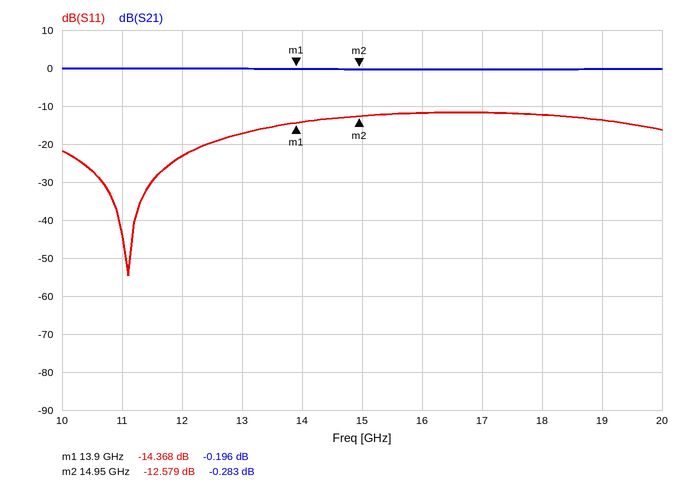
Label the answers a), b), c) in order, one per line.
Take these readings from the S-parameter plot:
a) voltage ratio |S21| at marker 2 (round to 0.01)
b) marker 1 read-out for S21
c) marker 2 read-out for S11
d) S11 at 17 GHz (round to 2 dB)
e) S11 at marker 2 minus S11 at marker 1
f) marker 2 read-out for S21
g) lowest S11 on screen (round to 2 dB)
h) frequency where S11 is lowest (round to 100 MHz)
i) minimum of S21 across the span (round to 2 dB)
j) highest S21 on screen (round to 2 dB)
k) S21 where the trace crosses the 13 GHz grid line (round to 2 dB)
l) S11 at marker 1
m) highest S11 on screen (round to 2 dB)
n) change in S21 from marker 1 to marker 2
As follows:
a) 0.97
b) -0.196 dB
c) -12.579 dB
d) -12 dB
e) 1.789 dB
f) -0.283 dB
g) -54 dB
h) 11.1 GHz
i) 0 dB
j) 0 dB
k) 0 dB
l) -14.368 dB
m) -12 dB
n) -0.087 dB
